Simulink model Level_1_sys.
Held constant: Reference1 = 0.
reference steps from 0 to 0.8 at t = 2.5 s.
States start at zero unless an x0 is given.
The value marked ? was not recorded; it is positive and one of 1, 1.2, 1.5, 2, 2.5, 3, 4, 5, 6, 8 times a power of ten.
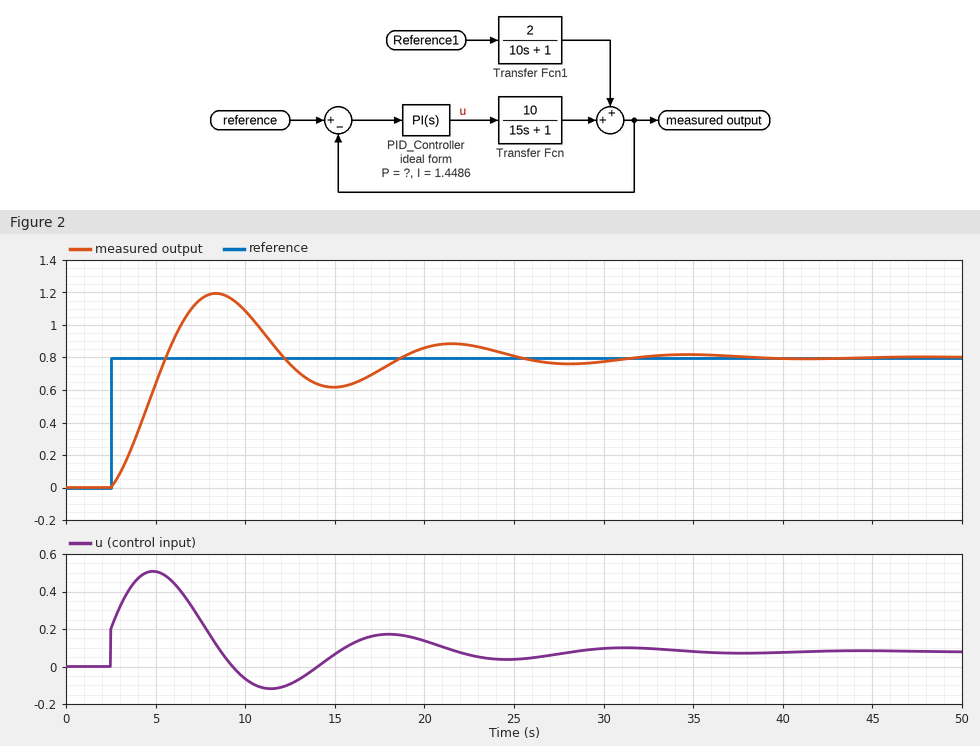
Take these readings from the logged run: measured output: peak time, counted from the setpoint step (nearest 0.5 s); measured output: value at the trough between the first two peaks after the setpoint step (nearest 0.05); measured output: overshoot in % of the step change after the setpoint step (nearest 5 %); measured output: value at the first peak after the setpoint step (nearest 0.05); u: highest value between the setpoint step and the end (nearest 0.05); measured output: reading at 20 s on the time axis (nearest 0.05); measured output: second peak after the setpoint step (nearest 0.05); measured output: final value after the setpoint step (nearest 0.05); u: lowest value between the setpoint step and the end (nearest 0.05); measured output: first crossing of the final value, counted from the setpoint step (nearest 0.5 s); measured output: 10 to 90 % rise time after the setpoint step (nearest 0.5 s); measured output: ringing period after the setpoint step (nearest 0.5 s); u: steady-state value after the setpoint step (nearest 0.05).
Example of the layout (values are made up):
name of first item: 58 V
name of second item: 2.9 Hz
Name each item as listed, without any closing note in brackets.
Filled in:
measured output: peak time, counted from the setpoint step: 6.0 s
measured output: value at the trough between the first two peaks after the setpoint step: 0.60
measured output: overshoot in % of the step change after the setpoint step: 50 %
measured output: value at the first peak after the setpoint step: 1.20
u: highest value between the setpoint step and the end: 0.50
measured output: reading at 20 s on the time axis: 0.85
measured output: second peak after the setpoint step: 0.90
measured output: final value after the setpoint step: 0.80
u: lowest value between the setpoint step and the end: -0.10
measured output: first crossing of the final value, counted from the setpoint step: 3.0 s
measured output: 10 to 90 % rise time after the setpoint step: 2.5 s
measured output: ringing period after the setpoint step: 13.0 s
u: steady-state value after the setpoint step: 0.10
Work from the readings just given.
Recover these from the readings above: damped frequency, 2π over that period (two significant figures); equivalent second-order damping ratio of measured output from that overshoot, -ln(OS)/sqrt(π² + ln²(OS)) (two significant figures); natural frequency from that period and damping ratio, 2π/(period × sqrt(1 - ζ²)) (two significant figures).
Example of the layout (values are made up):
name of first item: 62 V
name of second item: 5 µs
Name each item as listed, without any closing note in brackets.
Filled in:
damped frequency, 2π over that period: 0.48 rad/s
equivalent second-order damping ratio of measured output from that overshoot, -ln(OS)/sqrt(π² + ln²(OS)): 0.22
natural frequency from that period and damping ratio, 2π/(period × sqrt(1 - ζ²)): 0.50 rad/s
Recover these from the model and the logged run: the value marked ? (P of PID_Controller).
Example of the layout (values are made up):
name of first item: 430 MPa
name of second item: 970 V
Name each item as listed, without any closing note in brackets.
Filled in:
the value marked ?: 0.25
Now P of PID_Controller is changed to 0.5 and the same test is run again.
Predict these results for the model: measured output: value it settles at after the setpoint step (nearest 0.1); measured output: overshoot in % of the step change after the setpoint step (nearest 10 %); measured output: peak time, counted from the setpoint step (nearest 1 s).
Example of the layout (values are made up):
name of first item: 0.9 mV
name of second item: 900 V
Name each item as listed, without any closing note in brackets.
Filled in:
measured output: value it settles at after the setpoint step: 0.8
measured output: overshoot in % of the step change after the setpoint step: 40 %
measured output: peak time, counted from the setpoint step: 4 s
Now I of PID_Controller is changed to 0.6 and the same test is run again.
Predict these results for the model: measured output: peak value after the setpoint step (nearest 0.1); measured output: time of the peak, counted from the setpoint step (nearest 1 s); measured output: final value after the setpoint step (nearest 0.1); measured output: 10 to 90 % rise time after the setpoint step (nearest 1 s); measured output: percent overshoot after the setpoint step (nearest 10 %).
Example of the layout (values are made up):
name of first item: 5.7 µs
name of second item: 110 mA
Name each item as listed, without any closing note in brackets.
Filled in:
measured output: peak value after the setpoint step: 1.1
measured output: time of the peak, counted from the setpoint step: 9 s
measured output: final value after the setpoint step: 0.8
measured output: 10 to 90 % rise time after the setpoint step: 4 s
measured output: percent overshoot after the setpoint step: 30 %
